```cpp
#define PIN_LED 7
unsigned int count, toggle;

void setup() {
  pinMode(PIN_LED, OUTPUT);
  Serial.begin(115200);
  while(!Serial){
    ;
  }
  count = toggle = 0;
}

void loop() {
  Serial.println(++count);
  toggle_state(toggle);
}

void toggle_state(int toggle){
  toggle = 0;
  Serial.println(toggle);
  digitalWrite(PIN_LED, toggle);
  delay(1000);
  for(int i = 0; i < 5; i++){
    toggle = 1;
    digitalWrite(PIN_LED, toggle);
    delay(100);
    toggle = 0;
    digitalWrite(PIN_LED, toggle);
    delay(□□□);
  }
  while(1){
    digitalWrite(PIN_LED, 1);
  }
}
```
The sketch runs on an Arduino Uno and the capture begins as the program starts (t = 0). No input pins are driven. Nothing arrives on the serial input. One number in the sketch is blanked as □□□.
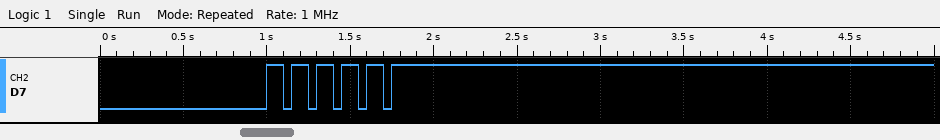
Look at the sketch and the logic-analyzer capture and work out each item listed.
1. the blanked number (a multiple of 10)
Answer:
50
